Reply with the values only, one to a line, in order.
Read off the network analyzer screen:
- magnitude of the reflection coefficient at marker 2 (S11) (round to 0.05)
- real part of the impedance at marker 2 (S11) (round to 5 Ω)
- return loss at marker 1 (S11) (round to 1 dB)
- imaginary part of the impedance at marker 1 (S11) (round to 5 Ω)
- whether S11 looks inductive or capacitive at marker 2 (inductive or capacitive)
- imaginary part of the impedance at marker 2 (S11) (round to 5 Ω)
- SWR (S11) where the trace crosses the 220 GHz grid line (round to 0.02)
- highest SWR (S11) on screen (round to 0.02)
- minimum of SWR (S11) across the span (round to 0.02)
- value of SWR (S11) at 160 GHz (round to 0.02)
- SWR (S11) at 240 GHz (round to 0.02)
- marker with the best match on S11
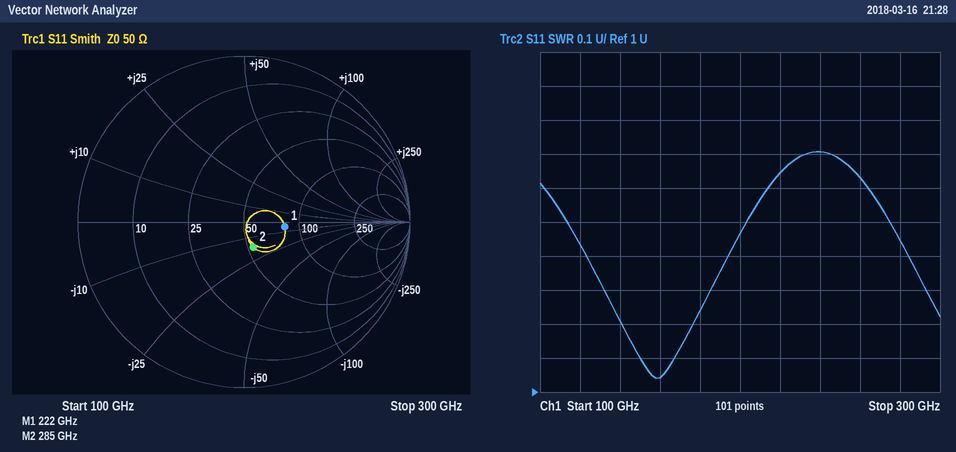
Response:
0.15
55 Ω
12 dB
-5 Ω
capacitive
-15 Ω
1.64
1.70
1.04
1.04
1.70
marker 2
